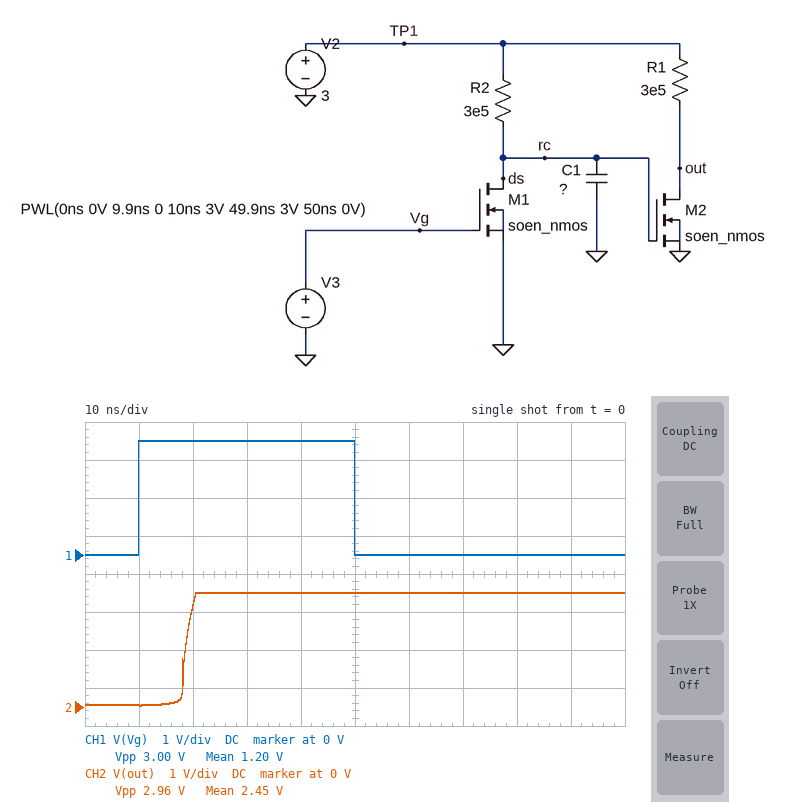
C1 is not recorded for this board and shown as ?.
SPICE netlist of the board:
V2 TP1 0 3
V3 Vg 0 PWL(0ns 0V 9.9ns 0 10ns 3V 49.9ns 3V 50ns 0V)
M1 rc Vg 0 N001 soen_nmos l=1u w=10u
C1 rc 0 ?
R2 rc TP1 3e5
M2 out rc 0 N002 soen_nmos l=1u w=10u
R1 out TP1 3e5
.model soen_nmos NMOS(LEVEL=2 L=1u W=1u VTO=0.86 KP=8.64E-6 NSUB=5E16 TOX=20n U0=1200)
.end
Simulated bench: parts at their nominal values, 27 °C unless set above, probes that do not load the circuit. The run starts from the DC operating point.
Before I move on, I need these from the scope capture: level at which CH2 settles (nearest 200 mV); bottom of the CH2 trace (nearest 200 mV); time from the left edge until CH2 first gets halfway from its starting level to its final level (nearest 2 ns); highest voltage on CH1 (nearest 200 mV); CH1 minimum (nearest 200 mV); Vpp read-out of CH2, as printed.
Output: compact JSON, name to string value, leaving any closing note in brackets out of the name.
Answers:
{"level at which CH2 settles": "3.0 V", "bottom of the CH2 trace": "0 V", "time from the left edge until CH2 first gets halfway from its starting level to its final level": "18 ns", "highest voltage on CH1": "3.0 V", "CH1 minimum": "0 V", "Vpp read-out of CH2, as printed": "2.96 V"}
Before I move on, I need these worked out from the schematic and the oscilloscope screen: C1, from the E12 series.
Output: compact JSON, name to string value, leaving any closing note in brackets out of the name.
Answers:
{"C1, from the E12 series": "820 fF"}
